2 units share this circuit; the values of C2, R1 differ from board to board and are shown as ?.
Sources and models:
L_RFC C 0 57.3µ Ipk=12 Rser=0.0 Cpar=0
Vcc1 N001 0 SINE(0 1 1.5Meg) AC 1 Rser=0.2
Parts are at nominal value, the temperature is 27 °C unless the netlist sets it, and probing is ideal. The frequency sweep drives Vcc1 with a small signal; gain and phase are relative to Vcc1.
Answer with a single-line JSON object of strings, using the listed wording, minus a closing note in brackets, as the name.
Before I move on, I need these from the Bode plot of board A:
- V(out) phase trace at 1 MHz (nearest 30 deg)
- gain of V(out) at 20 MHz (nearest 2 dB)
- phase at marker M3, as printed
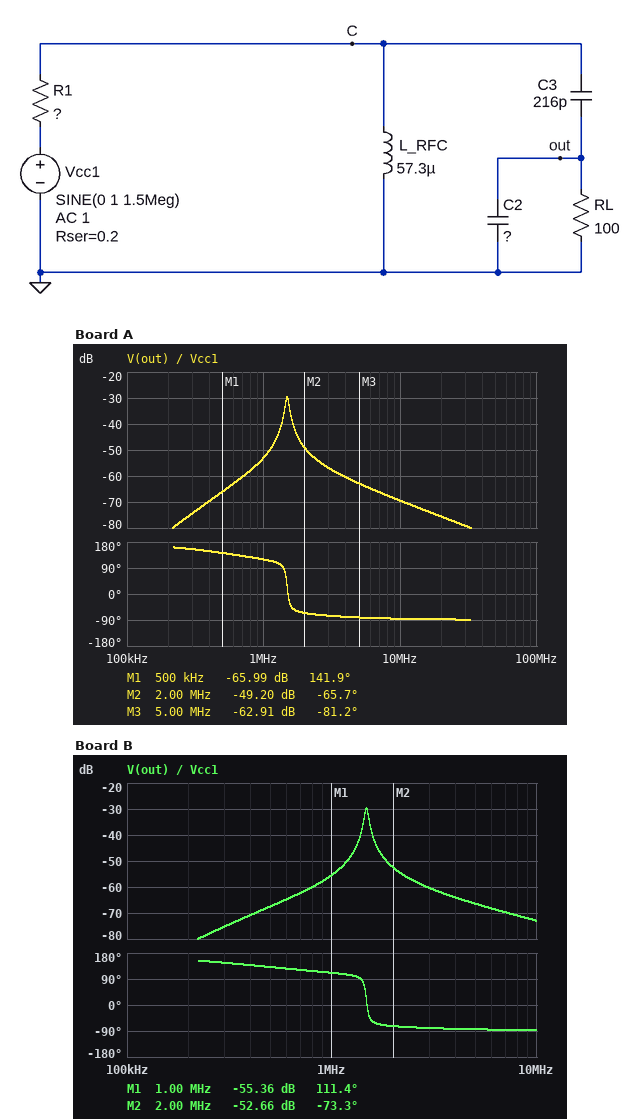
{"V(out) phase trace at 1 MHz": "120 deg", "gain of V(out) at 20 MHz": "-76 dB", "phase at marker M3, as printed": "-81.2 deg"}
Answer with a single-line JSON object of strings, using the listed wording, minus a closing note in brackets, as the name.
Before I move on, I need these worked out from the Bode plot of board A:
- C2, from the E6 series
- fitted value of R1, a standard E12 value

{"C2, from the E6 series": "2.2 nF", "fitted value of R1, a standard E12 value": "22 kΩ"}
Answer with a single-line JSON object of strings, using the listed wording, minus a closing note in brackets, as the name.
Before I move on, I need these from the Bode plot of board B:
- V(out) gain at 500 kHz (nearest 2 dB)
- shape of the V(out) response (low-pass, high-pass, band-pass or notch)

{"V(out) gain at 500 kHz": "-68 dB", "shape of the V(out) response": "band-pass"}
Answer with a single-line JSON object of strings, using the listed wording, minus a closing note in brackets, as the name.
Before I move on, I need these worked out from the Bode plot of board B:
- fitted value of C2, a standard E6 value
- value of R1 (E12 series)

{"fitted value of C2, a standard E6 value": "3.3 nF", "value of R1": "22 kΩ"}
